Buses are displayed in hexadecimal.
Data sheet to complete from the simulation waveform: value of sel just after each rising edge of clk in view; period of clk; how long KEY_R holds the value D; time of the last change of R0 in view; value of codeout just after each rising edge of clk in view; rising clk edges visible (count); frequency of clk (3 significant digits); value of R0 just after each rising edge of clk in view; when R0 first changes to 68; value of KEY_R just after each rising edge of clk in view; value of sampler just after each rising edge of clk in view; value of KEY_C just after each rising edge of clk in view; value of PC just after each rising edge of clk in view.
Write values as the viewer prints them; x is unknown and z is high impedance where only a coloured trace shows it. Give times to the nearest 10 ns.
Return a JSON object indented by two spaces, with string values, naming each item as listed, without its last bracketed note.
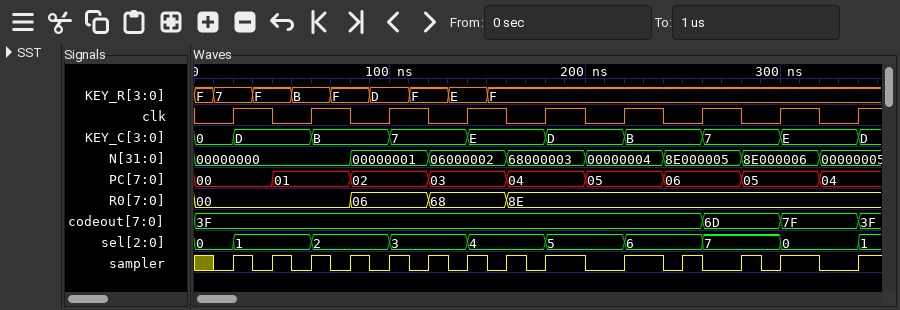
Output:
{
  "value of sel just after each rising edge of clk in view": "1, 2, 3, 4, 5, 6, 7, 0, 1",
  "period of clk": "40 ns",
  "how long KEY_R holds the value D": "20 ns",
  "time of the last change of R0 in view": "160 ns",
  "value of codeout just after each rising edge of clk in view": "3F, 3F, 3F, 3F, 3F, 3F, 6D, 7F, 3F",
  "rising clk edges visible": "9",
  "frequency of clk": "25.0 MHz",
  "value of R0 just after each rising edge of clk in view": "00, 00, 06, 68, 8E, 8E, 8E, 8E, 8E",
  "when R0 first changes to 68": "120 ns",
  "value of KEY_R just after each rising edge of clk in view": "7, B, D, E, F, F, F, F, F",
  "value of sampler just after each rising edge of clk in view": "1 1 1 1 1 1 0 1 1",
  "value of KEY_C just after each rising edge of clk in view": "D, B, 7, E, D, B, 7, E, D",
  "value of PC just after each rising edge of clk in view": "00, 01, 02, 03, 04, 05, 06, 05, 04"
}
